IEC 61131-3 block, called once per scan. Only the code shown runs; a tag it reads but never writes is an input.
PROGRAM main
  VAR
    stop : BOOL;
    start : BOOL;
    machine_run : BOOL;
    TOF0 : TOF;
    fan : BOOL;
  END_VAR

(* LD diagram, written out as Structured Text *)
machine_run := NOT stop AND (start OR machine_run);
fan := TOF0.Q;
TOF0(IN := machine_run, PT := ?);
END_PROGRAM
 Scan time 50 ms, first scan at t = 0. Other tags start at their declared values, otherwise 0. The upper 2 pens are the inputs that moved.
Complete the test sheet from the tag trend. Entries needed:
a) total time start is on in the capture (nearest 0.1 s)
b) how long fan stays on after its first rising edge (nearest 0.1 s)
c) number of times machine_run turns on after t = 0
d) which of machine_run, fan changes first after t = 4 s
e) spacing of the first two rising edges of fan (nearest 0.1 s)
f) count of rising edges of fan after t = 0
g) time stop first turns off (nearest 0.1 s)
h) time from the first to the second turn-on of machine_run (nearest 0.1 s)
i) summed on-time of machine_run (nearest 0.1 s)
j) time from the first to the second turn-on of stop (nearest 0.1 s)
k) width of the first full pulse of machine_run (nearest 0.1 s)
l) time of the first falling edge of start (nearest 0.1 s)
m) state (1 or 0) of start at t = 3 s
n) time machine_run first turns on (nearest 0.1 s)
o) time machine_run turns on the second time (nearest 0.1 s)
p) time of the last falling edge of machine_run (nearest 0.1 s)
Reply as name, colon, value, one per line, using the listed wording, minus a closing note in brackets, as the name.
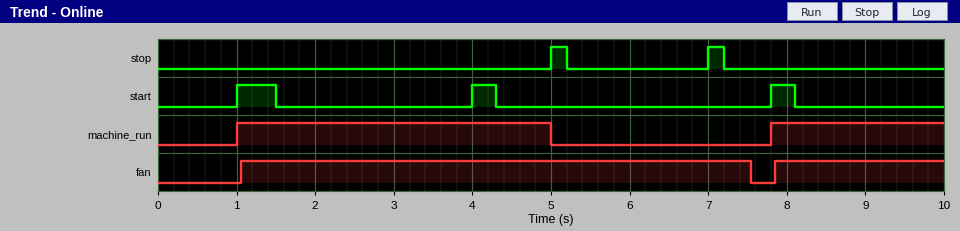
total time start is on in the capture: 1.1 s
how long fan stays on after its first rising edge: 6.5 s
number of times machine_run turns on after t = 0: 2
which of machine_run, fan changes first after t = 4 s: machine_run
spacing of the first two rising edges of fan: 6.8 s
count of rising edges of fan after t = 0: 2
time stop first turns off: 5.2 s
time from the first to the second turn-on of machine_run: 6.8 s
summed on-time of machine_run: 6.2 s
time from the first to the second turn-on of stop: 2.0 s
width of the first full pulse of machine_run: 4.0 s
time of the first falling edge of start: 1.5 s
state (1 or 0) of start at t = 3 s: 0
time machine_run first turns on: 1.0 s
time machine_run turns on the second time: 7.8 s
time of the last falling edge of machine_run: 5.0 s
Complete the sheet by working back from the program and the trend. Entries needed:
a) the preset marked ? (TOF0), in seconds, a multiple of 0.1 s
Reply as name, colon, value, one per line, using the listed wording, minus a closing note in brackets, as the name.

the preset marked ? (TOF0), in seconds, a multiple of 0.1 s: 2.5 s
